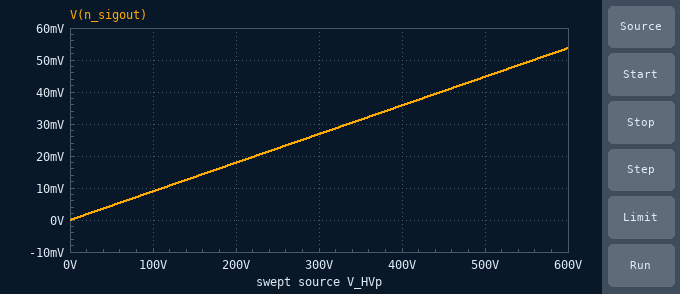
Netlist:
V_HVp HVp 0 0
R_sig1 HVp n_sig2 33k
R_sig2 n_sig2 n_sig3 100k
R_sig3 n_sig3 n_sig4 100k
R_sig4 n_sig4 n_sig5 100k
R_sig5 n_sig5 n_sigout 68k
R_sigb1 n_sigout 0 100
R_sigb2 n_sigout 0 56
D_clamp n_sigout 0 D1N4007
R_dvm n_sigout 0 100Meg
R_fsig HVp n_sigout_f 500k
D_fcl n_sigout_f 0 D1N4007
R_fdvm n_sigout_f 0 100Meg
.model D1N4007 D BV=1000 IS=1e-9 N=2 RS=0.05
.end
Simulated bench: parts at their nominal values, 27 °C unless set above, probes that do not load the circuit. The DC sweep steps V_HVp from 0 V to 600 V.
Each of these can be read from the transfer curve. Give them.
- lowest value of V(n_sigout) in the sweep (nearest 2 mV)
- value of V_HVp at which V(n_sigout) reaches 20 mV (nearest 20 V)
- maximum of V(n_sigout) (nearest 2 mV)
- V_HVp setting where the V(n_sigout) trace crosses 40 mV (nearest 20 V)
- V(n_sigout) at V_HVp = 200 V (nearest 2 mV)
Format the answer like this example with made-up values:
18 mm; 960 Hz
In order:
0 V; 220 V; 54 mV; 440 V; 18 mV
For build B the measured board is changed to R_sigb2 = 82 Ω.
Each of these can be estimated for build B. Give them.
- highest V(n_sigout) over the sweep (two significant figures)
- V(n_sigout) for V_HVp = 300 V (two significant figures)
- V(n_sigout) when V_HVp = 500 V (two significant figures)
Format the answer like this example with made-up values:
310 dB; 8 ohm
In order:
67 mV; 34 mV; 56 mV
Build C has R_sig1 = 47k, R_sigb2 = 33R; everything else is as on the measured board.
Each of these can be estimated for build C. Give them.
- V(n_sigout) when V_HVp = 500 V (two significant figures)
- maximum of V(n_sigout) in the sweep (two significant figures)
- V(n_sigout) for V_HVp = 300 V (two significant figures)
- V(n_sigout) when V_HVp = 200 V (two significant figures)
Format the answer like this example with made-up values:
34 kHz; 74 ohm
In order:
30 mV; 36 mV; 18 mV; 12 mV
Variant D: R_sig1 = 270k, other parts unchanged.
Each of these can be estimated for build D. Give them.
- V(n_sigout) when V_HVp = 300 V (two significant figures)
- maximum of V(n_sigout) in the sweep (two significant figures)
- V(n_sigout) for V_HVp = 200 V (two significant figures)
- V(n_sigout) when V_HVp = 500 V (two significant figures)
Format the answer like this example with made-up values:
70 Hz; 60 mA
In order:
17 mV; 34 mV; 11 mV; 28 mV
